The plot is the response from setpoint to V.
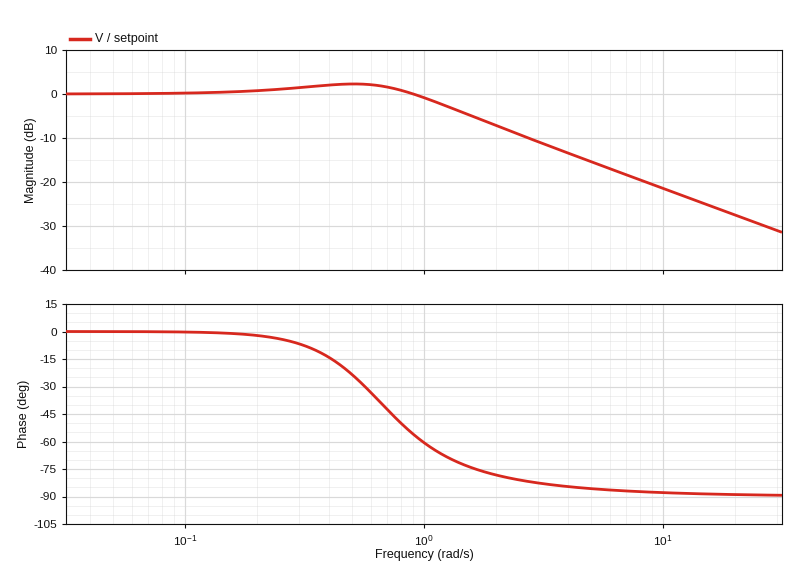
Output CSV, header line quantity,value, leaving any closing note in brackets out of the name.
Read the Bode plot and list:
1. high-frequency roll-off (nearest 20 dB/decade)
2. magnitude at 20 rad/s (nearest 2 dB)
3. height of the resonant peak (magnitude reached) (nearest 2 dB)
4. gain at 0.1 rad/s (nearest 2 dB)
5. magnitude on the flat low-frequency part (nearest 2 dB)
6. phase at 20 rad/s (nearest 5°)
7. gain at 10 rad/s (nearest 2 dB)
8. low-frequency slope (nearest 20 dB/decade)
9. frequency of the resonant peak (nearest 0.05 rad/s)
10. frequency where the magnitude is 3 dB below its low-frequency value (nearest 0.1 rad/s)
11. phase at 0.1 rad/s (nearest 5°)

quantity,value
high-frequency roll-off,-20 dB/decade
magnitude at 20 rad/s,-28 dB
height of the resonant peak (magnitude reached),2 dB
gain at 0.1 rad/s,0 dB
magnitude on the flat low-frequency part,0 dB
phase at 20 rad/s,-90°
gain at 10 rad/s,-22 dB
low-frequency slope,0 dB/decade
frequency of the resonant peak,0.50 rad/s
frequency where the magnitude is 3 dB below its low-frequency value,1.3 rad/s
phase at 0.1 rad/s,0°
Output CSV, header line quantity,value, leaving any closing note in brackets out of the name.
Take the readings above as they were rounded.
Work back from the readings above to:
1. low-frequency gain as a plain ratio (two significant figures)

quantity,value
low-frequency gain as a plain ratio,1.0
